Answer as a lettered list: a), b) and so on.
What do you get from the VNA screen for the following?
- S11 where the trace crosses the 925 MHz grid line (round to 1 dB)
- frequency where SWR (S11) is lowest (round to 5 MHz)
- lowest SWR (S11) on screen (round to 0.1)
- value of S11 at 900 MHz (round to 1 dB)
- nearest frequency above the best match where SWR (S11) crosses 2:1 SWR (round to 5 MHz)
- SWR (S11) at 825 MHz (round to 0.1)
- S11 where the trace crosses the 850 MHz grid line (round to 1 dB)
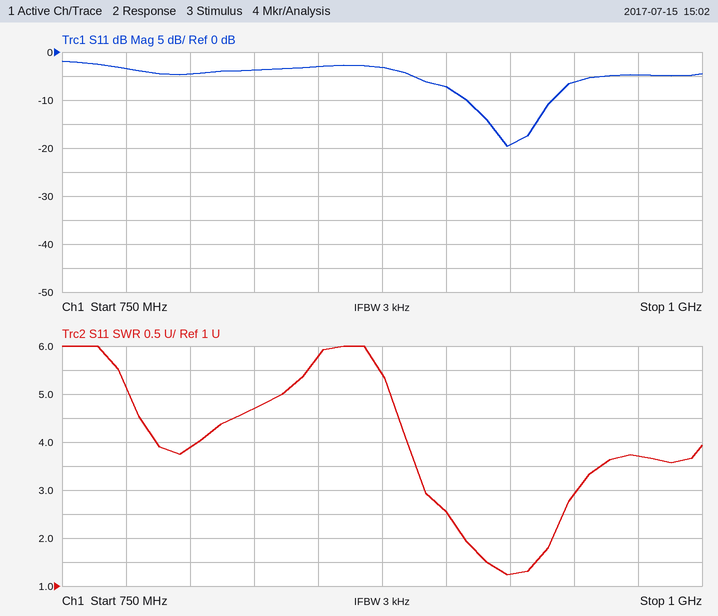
a) -19 dB
b) 925 MHz
c) 1.2
d) -7 dB
e) 940 MHz
f) 4.7
g) -3 dB
